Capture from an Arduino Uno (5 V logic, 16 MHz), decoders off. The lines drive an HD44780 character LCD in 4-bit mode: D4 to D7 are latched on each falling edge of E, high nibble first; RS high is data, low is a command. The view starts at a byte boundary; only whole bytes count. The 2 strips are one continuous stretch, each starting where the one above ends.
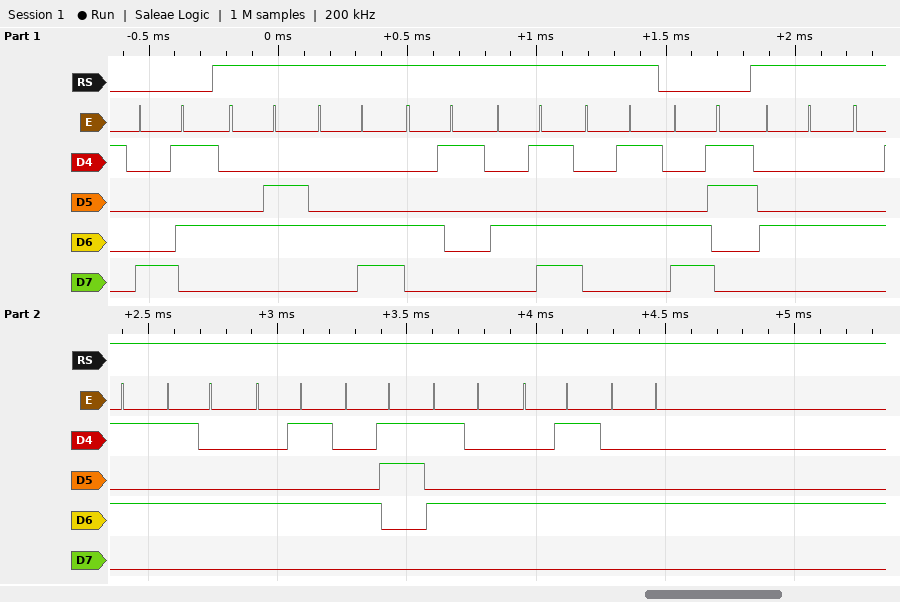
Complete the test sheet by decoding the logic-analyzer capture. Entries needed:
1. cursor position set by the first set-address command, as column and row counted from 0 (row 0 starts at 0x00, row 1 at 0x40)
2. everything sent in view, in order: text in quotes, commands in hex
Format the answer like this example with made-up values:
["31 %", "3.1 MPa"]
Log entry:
["column 5, row 0", "0x85 \"FLAME\" 0xC3 \"DETECTED\""]
